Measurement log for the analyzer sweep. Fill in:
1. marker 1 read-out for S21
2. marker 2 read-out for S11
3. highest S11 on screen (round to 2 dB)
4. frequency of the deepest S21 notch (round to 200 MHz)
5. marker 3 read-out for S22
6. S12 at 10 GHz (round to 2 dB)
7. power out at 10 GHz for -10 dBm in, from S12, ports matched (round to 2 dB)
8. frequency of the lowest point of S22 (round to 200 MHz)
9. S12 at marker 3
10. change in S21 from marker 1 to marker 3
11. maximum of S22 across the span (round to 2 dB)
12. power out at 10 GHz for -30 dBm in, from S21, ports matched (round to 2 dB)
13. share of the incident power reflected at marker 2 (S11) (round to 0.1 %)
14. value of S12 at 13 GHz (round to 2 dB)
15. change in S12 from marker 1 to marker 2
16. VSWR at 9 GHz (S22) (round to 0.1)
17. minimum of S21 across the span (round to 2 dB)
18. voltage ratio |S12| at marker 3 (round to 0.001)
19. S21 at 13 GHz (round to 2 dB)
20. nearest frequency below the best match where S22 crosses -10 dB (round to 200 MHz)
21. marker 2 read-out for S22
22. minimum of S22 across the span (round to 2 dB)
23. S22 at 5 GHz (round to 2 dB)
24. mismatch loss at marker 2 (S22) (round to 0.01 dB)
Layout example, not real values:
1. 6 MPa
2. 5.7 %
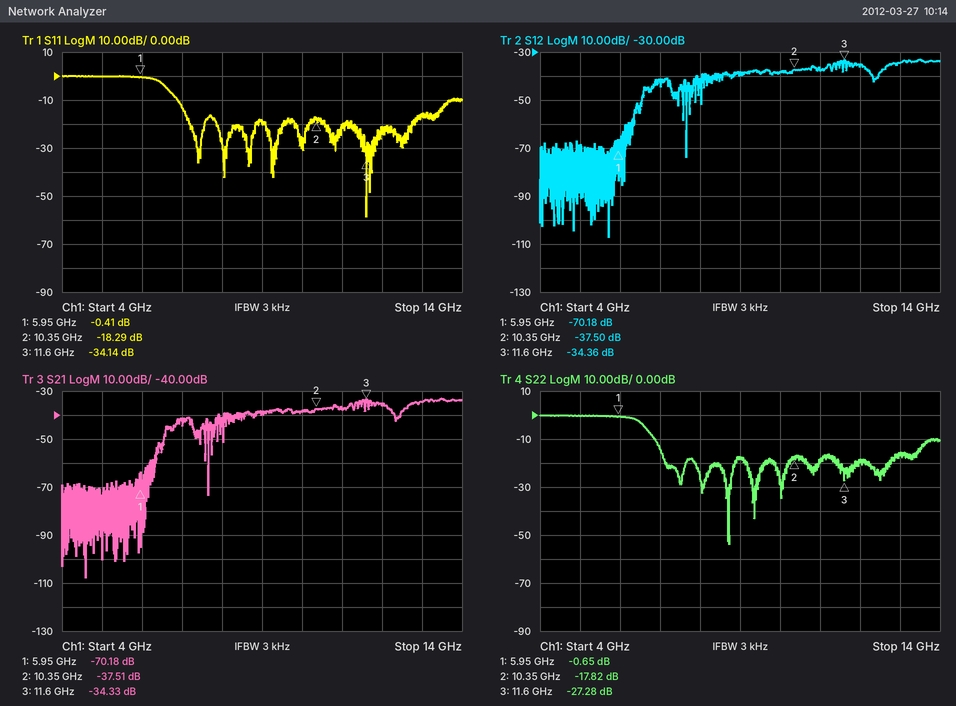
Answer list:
1. -70.18 dB
2. -18.29 dB
3. 0 dB
4. 4.6 GHz
5. -27.28 dB
6. -38 dB
7. -48 dBm
8. 8.8 GHz
9. -34.36 dB
10. 35.85 dB
11. 0 dB
12. -68 dBm
13. 1.5 %
14. -34 dB
15. 32.68 dB
16. 1.3
17. -108 dB
18. 0.019
19. -34 dB
20. 6.8 GHz
21. -17.82 dB
22. -54 dB
23. 0 dB
24. 0.07 dB
